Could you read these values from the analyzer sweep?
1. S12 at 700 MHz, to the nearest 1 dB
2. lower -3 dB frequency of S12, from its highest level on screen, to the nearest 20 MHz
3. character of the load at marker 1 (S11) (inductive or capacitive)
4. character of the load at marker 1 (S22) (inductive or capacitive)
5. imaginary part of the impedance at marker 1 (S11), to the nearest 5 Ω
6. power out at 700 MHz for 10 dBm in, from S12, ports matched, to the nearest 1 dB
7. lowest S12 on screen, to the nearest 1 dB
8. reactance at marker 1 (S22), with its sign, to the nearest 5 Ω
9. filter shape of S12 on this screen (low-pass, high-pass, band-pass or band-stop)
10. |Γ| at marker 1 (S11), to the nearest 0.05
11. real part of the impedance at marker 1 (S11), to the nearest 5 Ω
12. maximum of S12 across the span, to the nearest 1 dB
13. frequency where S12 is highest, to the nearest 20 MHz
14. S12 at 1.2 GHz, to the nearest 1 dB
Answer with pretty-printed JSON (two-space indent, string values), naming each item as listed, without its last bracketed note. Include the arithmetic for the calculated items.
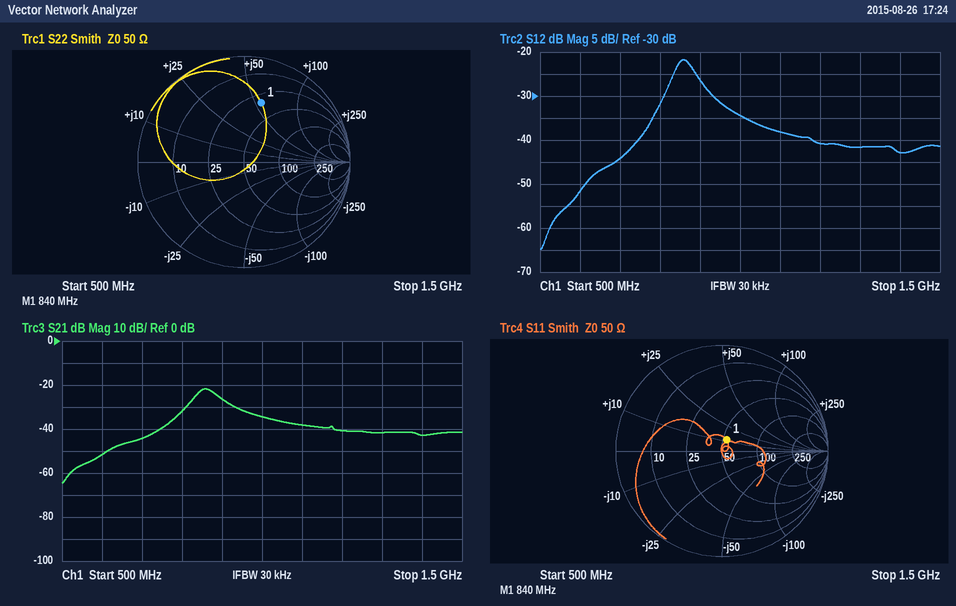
{
  "S12 at 700 MHz, to the nearest 1 dB": "-44 dB",
  "lower -3 dB frequency of S12, from its highest level on screen, to the nearest 20 MHz": "840 MHz",
  "character of the load at marker 1 (S11)": "inductive",
  "character of the load at marker 1 (S22)": "inductive",
  "imaginary part of the impedance at marker 1 (S11), to the nearest 5 Ω": "+10 Ω",
  "power out at 700 MHz for 10 dBm in, from S12, ports matched, to the nearest 1 dB": "10 dBm + (-44 dB) = -34 dBm",
  "lowest S12 on screen, to the nearest 1 dB": "-65 dB",
  "reactance at marker 1 (S22), with its sign, to the nearest 5 Ω": "+55 Ω",
  "filter shape of S12 on this screen": "band-pass",
  "|Γ| at marker 1 (S11), to the nearest 0.05": "0.10",
  "real part of the impedance at marker 1 (S11), to the nearest 5 Ω": "55 Ω",
  "maximum of S12 across the span, to the nearest 1 dB": "-22 dB",
  "frequency where S12 is highest, to the nearest 20 MHz": "860 MHz",
  "S12 at 1.2 GHz, to the nearest 1 dB": "-41 dB"
}
